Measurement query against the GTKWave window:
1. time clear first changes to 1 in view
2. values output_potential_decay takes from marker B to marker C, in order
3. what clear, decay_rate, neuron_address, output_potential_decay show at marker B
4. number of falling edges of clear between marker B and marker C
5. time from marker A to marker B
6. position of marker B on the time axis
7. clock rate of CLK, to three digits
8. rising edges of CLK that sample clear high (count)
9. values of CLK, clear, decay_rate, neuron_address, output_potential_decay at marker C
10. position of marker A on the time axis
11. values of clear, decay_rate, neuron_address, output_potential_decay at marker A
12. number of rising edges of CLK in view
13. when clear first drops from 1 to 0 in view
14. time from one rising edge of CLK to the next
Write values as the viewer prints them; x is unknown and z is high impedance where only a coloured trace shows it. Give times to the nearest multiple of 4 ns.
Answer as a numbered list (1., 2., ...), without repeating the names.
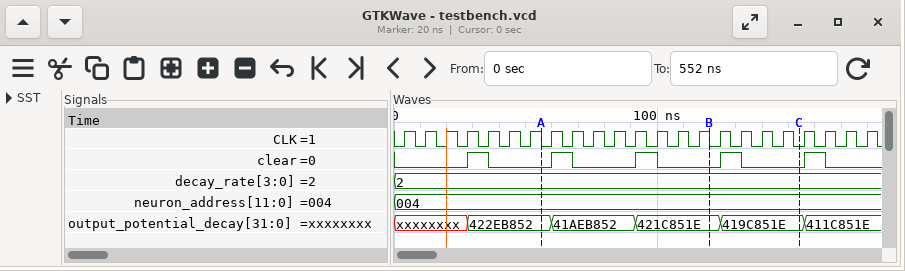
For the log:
1. 28 ns
2. 421C851E, 419C851E
3. clear=0, decay_rate=2, neuron_address=004, output_potential_decay=421C851E
4. 1
5. 64 ns
6. 120 ns
7. 125 MHz
8. 5
9. CLK=0, clear=0, decay_rate=2, neuron_address=004, output_potential_decay=419C851E
10. 56 ns
11. clear=0, decay_rate=2, neuron_address=004, output_potential_decay=422EB852
12. 23
13. 36 ns
14. 8 ns
